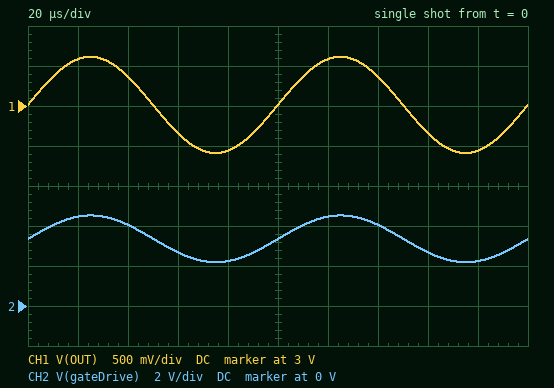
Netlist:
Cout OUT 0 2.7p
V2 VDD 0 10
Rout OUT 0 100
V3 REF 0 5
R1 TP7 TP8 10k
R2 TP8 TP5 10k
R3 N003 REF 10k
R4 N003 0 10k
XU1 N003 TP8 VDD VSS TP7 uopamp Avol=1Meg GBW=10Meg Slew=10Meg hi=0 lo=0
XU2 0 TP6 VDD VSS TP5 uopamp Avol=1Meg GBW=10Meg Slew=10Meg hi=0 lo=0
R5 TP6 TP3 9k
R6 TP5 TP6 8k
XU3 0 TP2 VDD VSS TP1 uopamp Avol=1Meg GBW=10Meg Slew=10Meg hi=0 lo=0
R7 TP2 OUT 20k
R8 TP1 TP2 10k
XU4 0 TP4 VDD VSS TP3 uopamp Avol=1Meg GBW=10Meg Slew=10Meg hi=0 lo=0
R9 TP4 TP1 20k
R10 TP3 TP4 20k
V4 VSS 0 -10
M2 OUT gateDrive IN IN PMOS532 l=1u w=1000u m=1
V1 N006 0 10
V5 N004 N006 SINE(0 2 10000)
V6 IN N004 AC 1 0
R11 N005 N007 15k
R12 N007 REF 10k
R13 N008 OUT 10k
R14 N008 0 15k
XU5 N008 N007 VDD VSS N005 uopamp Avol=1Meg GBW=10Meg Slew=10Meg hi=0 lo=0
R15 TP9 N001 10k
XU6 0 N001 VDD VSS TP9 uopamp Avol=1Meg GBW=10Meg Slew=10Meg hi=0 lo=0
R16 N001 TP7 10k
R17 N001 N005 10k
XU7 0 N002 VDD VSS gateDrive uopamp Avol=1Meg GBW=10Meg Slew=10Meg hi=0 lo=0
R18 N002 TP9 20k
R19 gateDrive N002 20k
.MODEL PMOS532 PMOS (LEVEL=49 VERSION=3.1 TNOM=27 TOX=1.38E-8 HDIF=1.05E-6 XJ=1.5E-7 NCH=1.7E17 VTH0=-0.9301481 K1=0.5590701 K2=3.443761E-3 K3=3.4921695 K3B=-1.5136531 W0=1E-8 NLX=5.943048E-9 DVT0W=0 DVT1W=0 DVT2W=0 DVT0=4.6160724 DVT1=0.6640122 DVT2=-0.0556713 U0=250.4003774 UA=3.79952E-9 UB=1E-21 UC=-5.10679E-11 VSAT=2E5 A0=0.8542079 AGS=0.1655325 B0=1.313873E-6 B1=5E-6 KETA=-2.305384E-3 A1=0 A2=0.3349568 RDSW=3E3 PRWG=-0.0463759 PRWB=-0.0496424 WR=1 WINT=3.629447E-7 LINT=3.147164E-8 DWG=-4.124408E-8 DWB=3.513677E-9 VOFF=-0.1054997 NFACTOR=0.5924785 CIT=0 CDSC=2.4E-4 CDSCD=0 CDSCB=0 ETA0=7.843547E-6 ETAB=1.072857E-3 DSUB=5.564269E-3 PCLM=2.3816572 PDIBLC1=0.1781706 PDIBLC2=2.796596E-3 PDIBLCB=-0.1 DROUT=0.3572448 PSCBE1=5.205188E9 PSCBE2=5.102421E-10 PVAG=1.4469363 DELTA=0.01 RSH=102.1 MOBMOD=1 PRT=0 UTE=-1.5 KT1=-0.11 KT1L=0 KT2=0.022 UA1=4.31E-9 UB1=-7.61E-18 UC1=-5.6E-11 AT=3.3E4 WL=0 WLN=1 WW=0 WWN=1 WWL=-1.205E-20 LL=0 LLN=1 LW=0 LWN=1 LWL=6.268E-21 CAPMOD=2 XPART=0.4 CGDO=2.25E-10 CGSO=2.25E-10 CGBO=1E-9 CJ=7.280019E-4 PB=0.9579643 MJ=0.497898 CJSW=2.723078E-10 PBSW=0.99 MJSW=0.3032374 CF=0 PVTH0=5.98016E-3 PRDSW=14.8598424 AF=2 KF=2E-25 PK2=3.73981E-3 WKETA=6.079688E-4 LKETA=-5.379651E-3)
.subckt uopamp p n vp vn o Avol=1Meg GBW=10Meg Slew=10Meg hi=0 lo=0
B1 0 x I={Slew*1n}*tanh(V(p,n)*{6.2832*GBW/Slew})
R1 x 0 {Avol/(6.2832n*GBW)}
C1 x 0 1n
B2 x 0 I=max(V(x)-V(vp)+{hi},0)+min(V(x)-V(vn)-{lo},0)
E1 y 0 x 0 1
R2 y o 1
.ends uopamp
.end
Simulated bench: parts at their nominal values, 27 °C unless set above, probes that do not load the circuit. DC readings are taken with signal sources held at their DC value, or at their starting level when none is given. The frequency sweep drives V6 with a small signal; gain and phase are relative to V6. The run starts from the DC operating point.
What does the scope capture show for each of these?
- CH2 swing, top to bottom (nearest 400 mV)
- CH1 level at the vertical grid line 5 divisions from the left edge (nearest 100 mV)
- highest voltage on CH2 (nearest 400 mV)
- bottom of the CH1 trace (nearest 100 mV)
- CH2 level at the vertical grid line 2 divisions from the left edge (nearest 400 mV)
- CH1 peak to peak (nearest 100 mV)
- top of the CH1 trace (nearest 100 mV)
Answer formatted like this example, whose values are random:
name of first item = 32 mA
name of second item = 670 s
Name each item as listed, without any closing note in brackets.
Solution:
CH2 swing, top to bottom = 2.4 V
CH1 level at the vertical grid line 5 divisions from the left edge = 3.0 V
highest voltage on CH2 = 4.4 V
bottom of the CH1 trace = 2.4 V
CH2 level at the vertical grid line 2 divisions from the left edge = 4.0 V
CH1 peak to peak = 1.2 V
top of the CH1 trace = 3.6 V
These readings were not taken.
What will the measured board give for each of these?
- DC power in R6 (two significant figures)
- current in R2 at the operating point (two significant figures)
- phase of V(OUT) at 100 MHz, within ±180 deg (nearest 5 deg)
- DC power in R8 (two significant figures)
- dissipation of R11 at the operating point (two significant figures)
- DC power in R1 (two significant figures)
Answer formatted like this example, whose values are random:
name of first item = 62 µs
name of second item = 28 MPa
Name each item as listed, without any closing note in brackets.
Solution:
DC power in R6 = 220 µW
current in R2 at the operating point = 380 µA
phase of V(OUT) at 100 MHz, within ±180 deg = -10 deg
DC power in R8 = 230 µW
dissipation of R11 at the operating point = 1.5 mW
DC power in R1 = 1.5 mW
